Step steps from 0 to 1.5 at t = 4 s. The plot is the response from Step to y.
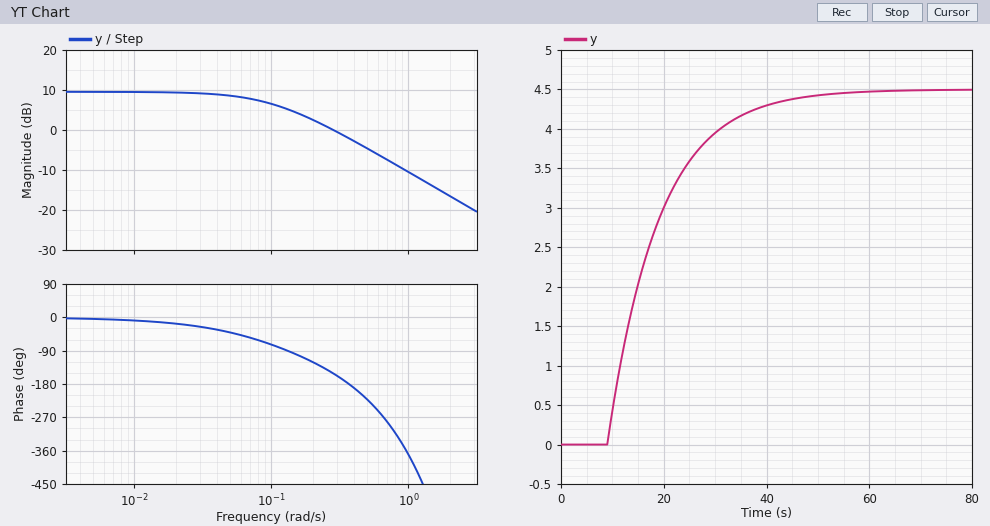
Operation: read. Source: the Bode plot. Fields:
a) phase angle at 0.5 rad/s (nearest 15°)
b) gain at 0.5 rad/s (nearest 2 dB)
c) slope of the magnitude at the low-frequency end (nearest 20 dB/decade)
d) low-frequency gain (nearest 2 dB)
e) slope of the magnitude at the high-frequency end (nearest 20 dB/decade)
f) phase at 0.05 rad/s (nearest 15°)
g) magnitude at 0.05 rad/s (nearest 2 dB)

-225°
-4 dB
0 dB/decade
10 dB
-20 dB/decade
-45°
8 dB
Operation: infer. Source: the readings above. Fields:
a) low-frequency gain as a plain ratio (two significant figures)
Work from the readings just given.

3.2
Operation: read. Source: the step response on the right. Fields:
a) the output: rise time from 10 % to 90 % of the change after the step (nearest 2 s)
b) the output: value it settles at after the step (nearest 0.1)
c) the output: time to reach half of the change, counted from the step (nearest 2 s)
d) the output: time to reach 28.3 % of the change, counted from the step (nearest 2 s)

22 s
4.5
12 s
8 s
